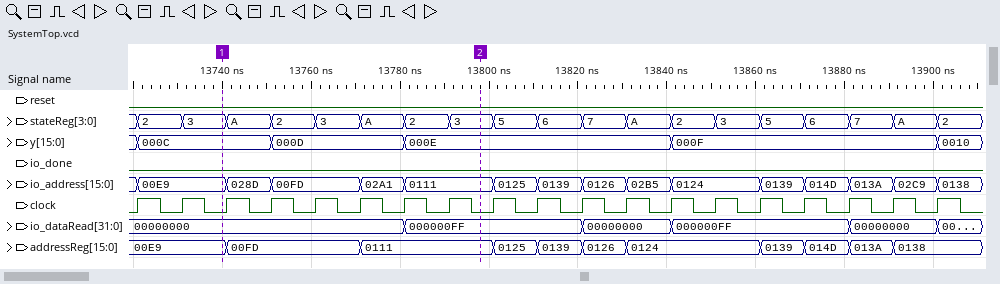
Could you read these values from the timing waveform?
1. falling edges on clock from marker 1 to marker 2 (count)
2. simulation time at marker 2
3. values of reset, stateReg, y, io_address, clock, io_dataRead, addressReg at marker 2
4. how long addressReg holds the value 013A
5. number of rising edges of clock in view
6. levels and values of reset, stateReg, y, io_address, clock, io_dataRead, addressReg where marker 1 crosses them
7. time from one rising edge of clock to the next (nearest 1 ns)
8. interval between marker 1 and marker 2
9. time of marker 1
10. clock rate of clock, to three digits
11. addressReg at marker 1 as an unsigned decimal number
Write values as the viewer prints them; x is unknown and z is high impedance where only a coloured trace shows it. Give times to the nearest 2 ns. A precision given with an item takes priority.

6
13798 ns
reset=0, stateReg=3, y=000E, io_address=0111, clock=0, io_dataRead=000000FF, addressReg=0111
10 ns
19
reset=0, stateReg=3, y=000C, io_address=00E9, clock=0, io_dataRead=00000000, addressReg=00E9
10 ns
58 ns
13740 ns
100 MHz
233
